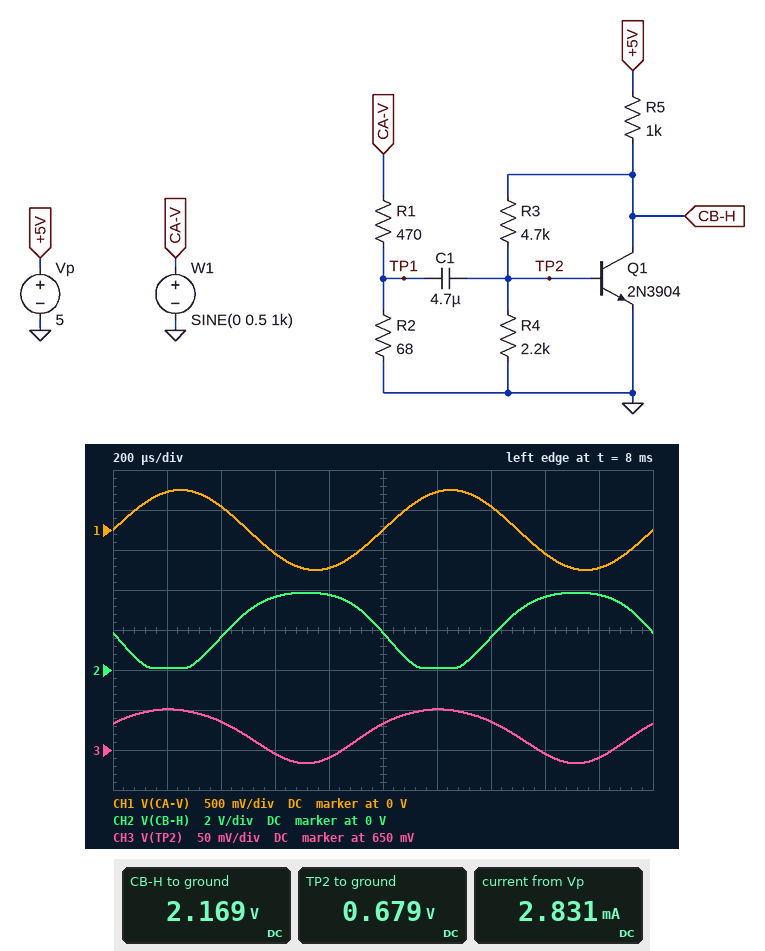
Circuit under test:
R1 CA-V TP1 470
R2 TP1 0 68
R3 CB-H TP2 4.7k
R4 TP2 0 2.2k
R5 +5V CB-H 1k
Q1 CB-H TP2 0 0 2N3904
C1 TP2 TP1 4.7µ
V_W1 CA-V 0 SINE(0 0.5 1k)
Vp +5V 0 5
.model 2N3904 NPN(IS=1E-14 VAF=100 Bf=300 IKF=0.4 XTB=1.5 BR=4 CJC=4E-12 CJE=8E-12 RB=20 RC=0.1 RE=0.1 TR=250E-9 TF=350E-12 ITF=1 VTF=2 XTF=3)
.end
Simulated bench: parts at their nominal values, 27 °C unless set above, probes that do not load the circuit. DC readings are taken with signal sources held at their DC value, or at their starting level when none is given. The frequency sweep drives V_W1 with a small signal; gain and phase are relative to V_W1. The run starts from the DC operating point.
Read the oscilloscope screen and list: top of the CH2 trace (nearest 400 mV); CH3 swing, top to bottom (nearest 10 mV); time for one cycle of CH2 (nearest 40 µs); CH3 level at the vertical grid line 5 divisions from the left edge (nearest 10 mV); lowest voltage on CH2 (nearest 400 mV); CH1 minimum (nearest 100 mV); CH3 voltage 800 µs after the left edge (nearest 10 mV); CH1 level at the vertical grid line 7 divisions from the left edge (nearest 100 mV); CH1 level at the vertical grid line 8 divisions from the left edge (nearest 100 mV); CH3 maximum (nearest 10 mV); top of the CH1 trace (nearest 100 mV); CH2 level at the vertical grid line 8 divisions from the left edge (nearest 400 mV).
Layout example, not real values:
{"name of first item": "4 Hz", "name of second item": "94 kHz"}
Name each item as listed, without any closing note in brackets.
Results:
{"top of the CH2 trace": "4.0 V", "CH3 swing, top to bottom": "70 mV", "time for one cycle of CH2": "1.00 ms", "CH3 level at the vertical grid line 5 divisions from the left edge": "680 mV", "lowest voltage on CH2": "0 V", "CH1 minimum": "-500 mV", "CH3 voltage 800 µs after the left edge": "640 mV", "CH1 level at the vertical grid line 7 divisions from the left edge": "300 mV", "CH1 level at the vertical grid line 8 divisions from the left edge": "-300 mV", "CH3 maximum": "700 mV", "top of the CH1 trace": "500 mV", "CH2 level at the vertical grid line 8 divisions from the left edge": "3.6 V"}
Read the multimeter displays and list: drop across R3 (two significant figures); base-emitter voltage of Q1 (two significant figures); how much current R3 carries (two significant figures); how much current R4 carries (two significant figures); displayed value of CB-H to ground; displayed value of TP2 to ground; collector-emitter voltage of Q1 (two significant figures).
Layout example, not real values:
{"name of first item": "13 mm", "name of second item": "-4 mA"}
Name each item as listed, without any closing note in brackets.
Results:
{"drop across R3": "1.5 V", "base-emitter voltage of Q1": "680 mV", "how much current R3 carries": "320 µA", "how much current R4 carries": "310 µA", "displayed value of CB-H to ground": "2.169 V", "displayed value of TP2 to ground": "0.679 V", "collector-emitter voltage of Q1": "2.2 V"}
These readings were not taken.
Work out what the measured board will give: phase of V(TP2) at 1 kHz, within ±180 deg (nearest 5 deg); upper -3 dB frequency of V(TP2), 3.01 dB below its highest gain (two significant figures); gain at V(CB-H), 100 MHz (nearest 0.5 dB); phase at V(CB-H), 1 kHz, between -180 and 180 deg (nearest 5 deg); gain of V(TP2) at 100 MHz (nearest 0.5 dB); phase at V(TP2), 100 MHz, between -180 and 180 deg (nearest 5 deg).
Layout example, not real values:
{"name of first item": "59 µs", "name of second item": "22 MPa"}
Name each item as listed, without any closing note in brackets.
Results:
{"phase of V(TP2) at 1 kHz, within ±180 deg": "15 deg", "upper -3 dB frequency of V(TP2), 3.01 dB below its highest gain": "35 MHz", "gain at V(CB-H), 100 MHz": "-3.5 dB", "phase at V(CB-H), 1 kHz, between -180 and 180 deg": "-165 deg", "gain of V(TP2) at 100 MHz": "-28.0 dB", "phase at V(TP2), 100 MHz, between -180 and 180 deg": "-5 deg"}
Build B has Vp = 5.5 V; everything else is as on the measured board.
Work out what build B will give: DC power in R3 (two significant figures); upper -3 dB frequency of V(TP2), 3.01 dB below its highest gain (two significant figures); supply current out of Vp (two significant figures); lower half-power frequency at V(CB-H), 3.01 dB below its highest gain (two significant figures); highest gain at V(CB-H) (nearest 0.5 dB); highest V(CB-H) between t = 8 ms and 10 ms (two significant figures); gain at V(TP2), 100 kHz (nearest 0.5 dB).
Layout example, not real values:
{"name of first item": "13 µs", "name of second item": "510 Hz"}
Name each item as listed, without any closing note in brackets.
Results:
{"DC power in R3": "480 µW", "upper -3 dB frequency of V(TP2), 3.01 dB below its highest gain": "50 MHz", "supply current out of Vp": "3.3 mA", "lower half-power frequency at V(CB-H), 3.01 dB below its highest gain": "310 Hz", "highest gain at V(CB-H)": "14.5 dB", "highest V(CB-H) between t = 8 ms and 10 ms": "4.1 V", "gain at V(TP2), 100 kHz": "-25.0 dB"}
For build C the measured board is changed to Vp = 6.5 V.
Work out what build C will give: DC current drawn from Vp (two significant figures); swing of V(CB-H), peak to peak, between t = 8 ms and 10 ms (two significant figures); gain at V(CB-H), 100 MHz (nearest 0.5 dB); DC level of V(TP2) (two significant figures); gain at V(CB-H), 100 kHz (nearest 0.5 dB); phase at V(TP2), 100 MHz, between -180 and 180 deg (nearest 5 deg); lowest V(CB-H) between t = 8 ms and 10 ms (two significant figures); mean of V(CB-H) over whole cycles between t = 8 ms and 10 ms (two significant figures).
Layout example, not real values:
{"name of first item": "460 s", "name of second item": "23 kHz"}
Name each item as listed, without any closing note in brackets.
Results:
{"DC current drawn from Vp": "4.3 mA", "swing of V(CB-H), peak to peak, between t = 8 ms and 10 ms": "4.5 V", "gain at V(CB-H), 100 MHz": "-3.0 dB", "DC level of V(TP2)": "690 mV", "gain at V(CB-H), 100 kHz": "15.5 dB", "phase at V(TP2), 100 MHz, between -180 and 180 deg": "-5 deg", "lowest V(CB-H) between t = 8 ms and 10 ms": "71 mV", "mean of V(CB-H) over whole cycles between t = 8 ms and 10 ms": "2.3 V"}
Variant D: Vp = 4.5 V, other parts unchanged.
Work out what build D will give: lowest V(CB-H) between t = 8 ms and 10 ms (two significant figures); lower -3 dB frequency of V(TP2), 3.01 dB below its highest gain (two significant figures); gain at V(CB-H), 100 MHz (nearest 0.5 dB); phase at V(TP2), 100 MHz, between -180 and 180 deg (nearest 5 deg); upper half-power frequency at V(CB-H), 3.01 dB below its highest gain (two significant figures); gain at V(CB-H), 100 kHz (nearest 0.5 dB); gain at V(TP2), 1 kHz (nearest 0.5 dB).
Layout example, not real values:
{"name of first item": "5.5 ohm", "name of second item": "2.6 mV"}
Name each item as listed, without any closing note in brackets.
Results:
{"lowest V(CB-H) between t = 8 ms and 10 ms": "100 mV", "lower -3 dB frequency of V(TP2), 3.01 dB below its highest gain": "260 Hz", "gain at V(CB-H), 100 MHz": "-4.0 dB", "phase at V(TP2), 100 MHz, between -180 and 180 deg": "-10 deg", "upper half-power frequency at V(CB-H), 3.01 dB below its highest gain": "15 MHz", "gain at V(CB-H), 100 kHz": "12.5 dB", "gain at V(TP2), 1 kHz": "-23.5 dB"}
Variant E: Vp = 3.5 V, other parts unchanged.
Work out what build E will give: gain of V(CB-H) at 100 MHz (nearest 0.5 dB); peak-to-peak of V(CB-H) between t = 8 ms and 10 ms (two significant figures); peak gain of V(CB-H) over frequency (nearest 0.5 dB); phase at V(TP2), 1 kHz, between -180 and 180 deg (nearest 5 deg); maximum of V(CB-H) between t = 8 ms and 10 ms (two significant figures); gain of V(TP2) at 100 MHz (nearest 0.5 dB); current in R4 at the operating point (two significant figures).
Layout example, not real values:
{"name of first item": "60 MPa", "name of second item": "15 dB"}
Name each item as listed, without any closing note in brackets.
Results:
{"gain of V(CB-H) at 100 MHz": "-5.0 dB", "peak-to-peak of V(CB-H) between t = 8 ms and 10 ms": "2.4 V", "peak gain of V(CB-H) over frequency": "9.5 dB", "phase at V(TP2), 1 kHz, between -180 and 180 deg": "10 deg", "maximum of V(CB-H) between t = 8 ms and 10 ms": "2.9 V", "gain of V(TP2) at 100 MHz": "-26.0 dB", "current in R4 at the operating point": "300 µA"}
